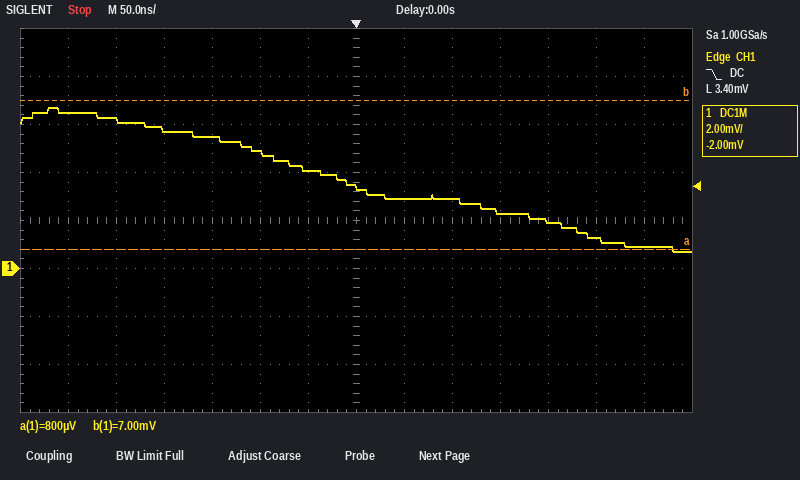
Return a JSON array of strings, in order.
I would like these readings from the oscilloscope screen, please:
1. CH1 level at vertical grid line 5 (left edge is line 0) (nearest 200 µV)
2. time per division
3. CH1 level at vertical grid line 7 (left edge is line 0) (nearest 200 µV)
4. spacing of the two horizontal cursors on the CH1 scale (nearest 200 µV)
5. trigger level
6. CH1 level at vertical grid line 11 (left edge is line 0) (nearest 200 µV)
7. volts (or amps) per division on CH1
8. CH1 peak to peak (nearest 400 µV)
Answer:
["4.8 mV", "50 ns", "3.4 mV", "6.2 mV", "3.40 mV", "2.0 mV", "2 mV", "6.0 mV"]
